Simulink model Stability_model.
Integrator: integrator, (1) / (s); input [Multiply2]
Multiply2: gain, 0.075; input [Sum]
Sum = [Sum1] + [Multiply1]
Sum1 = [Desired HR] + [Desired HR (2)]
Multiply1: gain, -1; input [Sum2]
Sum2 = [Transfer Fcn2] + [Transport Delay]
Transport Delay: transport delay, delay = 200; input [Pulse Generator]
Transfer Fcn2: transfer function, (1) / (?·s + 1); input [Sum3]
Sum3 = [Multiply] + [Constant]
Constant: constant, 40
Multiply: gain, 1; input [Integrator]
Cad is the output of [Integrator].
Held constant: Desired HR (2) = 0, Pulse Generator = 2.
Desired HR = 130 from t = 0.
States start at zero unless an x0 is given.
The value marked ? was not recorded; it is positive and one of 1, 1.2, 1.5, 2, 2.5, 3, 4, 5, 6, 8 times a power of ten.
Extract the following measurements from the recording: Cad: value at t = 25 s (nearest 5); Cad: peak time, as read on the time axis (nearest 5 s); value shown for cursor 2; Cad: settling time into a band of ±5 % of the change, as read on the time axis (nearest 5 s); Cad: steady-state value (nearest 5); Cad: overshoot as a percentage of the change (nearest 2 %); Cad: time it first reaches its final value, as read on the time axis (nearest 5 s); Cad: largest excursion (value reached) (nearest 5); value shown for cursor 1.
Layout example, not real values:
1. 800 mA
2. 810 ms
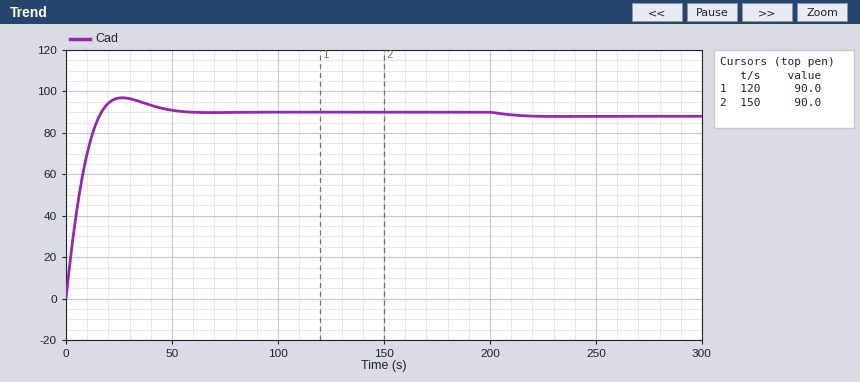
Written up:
1. 95
2. 25 s
3. 90.0
4. 45 s
5. 90
6. 10 %
7. 15 s
8. 95
9. 90.0
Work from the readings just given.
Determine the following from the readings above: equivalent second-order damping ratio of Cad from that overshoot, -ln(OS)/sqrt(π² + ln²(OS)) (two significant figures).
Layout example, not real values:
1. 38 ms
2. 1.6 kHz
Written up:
1. 0.59
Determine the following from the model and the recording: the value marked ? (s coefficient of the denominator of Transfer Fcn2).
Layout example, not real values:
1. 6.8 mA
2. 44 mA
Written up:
1. 6
